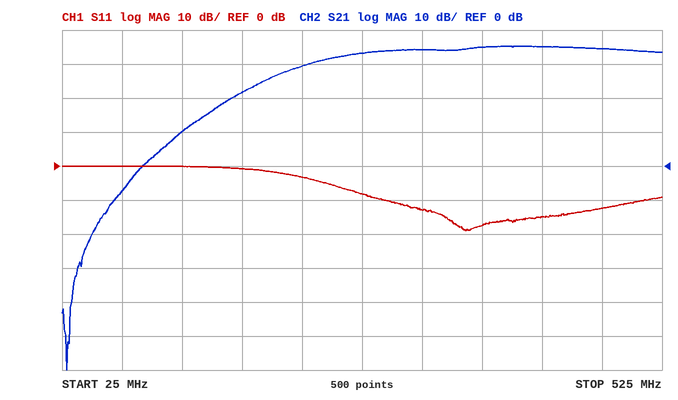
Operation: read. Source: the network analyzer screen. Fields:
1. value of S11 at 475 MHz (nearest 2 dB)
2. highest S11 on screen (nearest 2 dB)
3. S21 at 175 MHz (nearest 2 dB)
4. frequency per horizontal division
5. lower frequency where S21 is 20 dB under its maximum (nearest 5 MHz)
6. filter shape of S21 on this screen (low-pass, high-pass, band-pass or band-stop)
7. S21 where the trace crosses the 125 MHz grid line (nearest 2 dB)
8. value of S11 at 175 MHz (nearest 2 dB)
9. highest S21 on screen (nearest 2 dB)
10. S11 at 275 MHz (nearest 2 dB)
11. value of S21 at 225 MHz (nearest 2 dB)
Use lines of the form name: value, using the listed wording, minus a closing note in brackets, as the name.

value of S11 at 475 MHz: -12 dB
highest S11 on screen: 0 dB
S21 at 175 MHz: 22 dB
frequency per horizontal division: 50 MHz
lower frequency where S21 is 20 dB under its maximum: 145 MHz
filter shape of S21 on this screen: high-pass
S21 where the trace crosses the 125 MHz grid line: 10 dB
value of S11 at 175 MHz: 0 dB
highest S21 on screen: 36 dB
S11 at 275 MHz: -8 dB
value of S21 at 225 MHz: 30 dB
